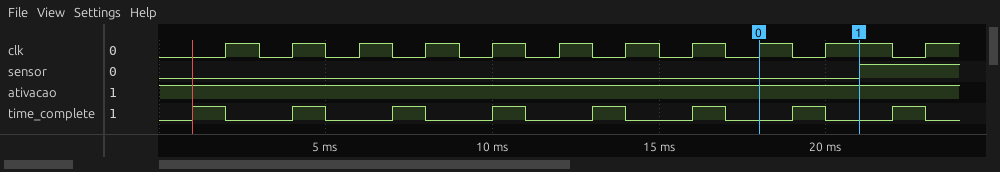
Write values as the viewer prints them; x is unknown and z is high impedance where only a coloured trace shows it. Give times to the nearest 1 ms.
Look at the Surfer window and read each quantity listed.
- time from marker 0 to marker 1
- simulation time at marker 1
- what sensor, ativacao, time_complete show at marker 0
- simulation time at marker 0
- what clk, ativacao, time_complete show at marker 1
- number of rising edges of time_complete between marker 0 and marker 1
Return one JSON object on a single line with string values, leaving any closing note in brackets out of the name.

{"time from marker 0 to marker 1": "3 ms", "simulation time at marker 1": "21 ms", "what sensor, ativacao, time_complete show at marker 0": "sensor=0, ativacao=1, time_complete=0", "simulation time at marker 0": "18 ms", "what clk, ativacao, time_complete show at marker 1": "clk=1, ativacao=1, time_complete=0", "number of rising edges of time_complete between marker 0 and marker 1": "1"}
